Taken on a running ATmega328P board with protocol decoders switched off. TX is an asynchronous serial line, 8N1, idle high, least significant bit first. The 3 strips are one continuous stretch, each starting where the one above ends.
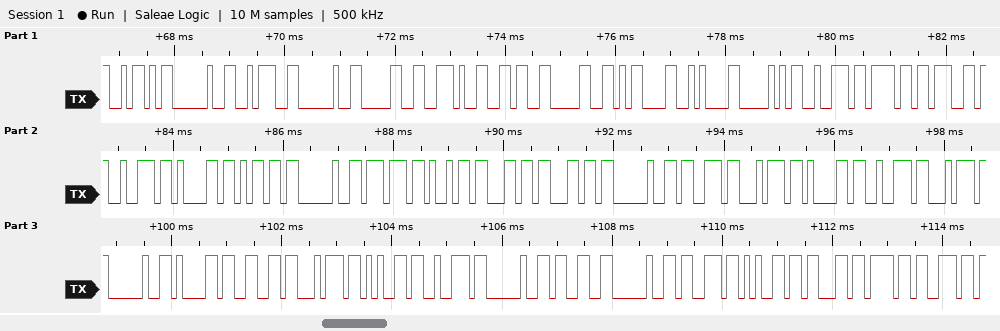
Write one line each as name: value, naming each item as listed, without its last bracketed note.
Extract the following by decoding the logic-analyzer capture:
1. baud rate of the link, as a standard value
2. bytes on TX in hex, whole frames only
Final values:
baud rate of the link, as a standard value: 9600 baud
bytes on TX in hex, whole frames only: 5A 20 3A 20 30 2E 36 30 0D 0A 50 72 6F 67 72 61 6D 20 77 69 6C 6C 20 73 74 61 72 74 20 61 66 74 65 72 20 33 20 73 65 63 6F 6E
